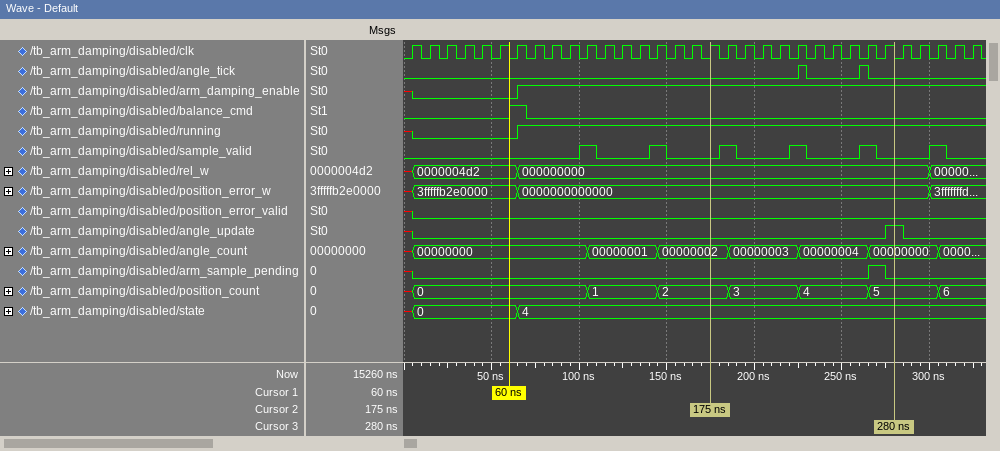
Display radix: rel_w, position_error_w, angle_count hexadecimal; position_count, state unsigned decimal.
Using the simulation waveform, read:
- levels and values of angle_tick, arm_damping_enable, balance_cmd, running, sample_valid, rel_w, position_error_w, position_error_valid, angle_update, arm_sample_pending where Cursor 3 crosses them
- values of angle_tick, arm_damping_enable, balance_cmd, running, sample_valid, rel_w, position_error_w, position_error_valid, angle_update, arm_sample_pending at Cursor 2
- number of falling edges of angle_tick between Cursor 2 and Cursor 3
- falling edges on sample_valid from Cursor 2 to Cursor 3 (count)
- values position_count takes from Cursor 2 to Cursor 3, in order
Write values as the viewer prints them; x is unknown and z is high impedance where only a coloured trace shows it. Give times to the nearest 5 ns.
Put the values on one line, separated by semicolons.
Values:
angle_tick=0, arm_damping_enable=1, balance_cmd=0, running=1, sample_valid=0, rel_w=000000000, position_error_w=0000000000000, position_error_valid=0, angle_update=1, arm_sample_pending=0; angle_tick=0, arm_damping_enable=1, balance_cmd=0, running=1, sample_valid=0, rel_w=000000000, position_error_w=0000000000000, position_error_valid=0, angle_update=0, arm_sample_pending=0; 2; 3; 2, 3, 4, 5
